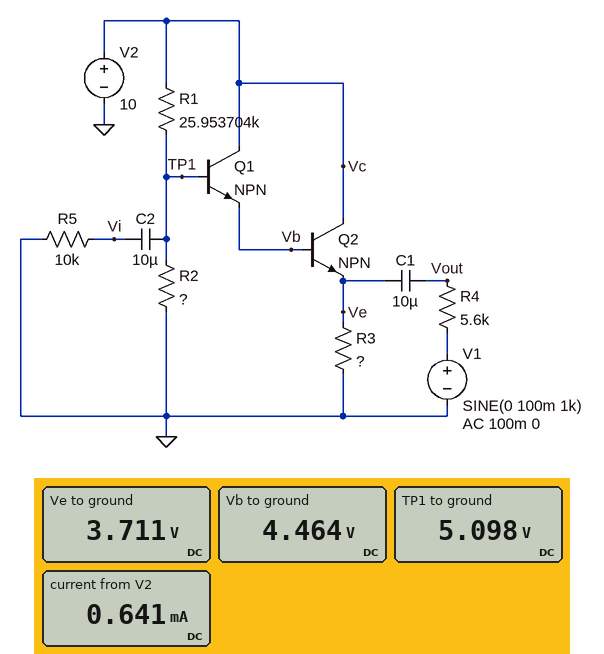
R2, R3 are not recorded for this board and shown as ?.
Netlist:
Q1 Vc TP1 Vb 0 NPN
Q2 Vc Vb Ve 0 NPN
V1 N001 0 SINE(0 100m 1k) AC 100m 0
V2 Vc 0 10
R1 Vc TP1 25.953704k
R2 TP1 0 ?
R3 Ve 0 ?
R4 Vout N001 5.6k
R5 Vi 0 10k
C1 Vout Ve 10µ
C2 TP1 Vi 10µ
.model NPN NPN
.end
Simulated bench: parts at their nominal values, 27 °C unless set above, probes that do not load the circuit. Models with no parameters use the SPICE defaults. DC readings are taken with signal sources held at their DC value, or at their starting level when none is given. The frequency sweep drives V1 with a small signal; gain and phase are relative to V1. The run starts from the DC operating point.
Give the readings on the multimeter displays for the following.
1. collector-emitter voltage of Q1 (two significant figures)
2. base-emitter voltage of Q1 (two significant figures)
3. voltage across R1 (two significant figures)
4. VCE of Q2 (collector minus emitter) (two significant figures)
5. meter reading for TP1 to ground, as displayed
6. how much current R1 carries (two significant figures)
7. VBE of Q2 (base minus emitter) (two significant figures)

5.5 V
630 mV
4.9 V
6.3 V
5.098 V
190 µA
750 mV
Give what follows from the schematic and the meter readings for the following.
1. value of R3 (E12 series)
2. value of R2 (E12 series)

8.2 kΩ
27 kΩ
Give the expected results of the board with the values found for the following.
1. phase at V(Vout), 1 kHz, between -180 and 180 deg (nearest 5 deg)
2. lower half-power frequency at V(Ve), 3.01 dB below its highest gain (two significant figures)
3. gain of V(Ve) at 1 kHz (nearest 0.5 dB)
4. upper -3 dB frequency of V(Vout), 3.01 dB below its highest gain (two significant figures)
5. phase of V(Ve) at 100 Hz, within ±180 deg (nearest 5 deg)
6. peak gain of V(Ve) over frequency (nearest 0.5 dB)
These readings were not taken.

-10 deg
2.8 Hz
-34.0 dB
2.8 Hz
0 deg
-34.0 dB
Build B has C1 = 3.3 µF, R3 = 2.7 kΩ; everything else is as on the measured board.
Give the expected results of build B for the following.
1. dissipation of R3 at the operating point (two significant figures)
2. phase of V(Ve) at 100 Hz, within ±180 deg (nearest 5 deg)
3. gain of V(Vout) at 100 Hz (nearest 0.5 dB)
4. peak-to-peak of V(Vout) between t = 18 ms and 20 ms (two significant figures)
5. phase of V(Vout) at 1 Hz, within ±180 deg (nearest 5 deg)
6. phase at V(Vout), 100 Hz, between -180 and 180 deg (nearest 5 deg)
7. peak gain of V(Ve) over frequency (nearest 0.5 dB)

4.9 mW
5 deg
-21.5 dB
2.2 mV
-5 deg
-80 deg
-43.5 dB
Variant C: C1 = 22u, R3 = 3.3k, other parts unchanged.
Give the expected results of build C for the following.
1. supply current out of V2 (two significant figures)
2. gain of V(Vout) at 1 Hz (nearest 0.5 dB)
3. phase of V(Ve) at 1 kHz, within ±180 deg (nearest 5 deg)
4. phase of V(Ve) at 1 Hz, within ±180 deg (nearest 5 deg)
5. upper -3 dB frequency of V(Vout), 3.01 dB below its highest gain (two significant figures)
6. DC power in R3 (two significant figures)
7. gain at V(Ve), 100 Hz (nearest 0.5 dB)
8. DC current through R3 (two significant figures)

1.3 mA
-2.0 dB
0 deg
50 deg
1.3 Hz
4.1 mW
-41.5 dB
1.1 mA
